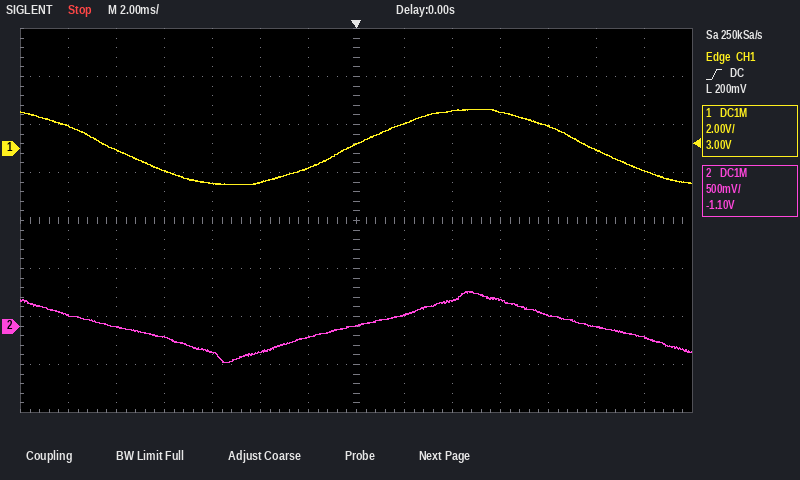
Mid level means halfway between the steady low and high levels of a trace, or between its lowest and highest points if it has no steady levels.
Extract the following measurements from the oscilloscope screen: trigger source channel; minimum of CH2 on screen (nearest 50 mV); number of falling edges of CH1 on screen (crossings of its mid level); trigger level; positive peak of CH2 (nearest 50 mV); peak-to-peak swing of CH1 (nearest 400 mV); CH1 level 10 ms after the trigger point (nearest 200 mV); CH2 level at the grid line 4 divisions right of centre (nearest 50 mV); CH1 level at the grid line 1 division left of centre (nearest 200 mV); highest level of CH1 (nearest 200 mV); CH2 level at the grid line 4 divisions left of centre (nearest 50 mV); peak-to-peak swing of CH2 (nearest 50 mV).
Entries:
CH1
-400 mV
2
200 mV
350 mV
3.2 V
0.0 V
100 mV
-800 mV
1.6 V
-100 mV
750 mV
